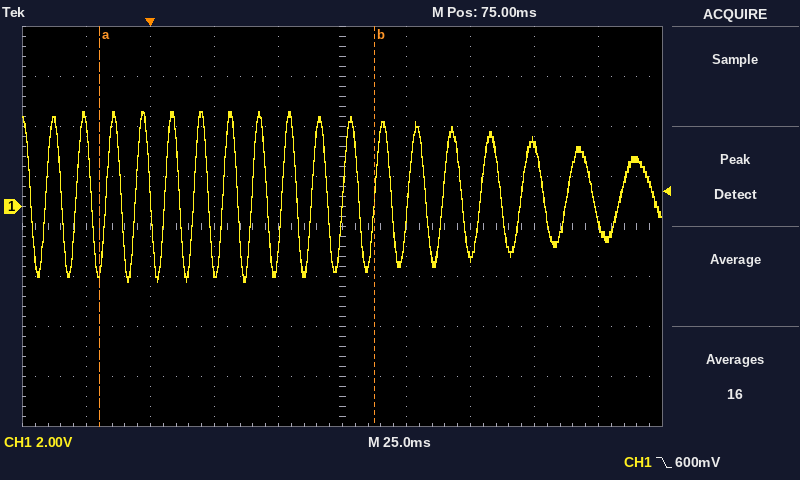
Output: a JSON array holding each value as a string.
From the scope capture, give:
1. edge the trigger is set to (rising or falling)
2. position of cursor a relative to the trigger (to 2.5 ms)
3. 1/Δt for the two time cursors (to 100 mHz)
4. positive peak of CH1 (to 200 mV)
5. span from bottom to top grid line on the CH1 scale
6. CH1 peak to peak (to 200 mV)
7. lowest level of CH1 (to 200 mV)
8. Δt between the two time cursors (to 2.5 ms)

["falling", "-20.0 ms", "9.3 Hz", "3.8 V", "16 V", "6.8 V", "-3.0 V", "107.5 ms"]
